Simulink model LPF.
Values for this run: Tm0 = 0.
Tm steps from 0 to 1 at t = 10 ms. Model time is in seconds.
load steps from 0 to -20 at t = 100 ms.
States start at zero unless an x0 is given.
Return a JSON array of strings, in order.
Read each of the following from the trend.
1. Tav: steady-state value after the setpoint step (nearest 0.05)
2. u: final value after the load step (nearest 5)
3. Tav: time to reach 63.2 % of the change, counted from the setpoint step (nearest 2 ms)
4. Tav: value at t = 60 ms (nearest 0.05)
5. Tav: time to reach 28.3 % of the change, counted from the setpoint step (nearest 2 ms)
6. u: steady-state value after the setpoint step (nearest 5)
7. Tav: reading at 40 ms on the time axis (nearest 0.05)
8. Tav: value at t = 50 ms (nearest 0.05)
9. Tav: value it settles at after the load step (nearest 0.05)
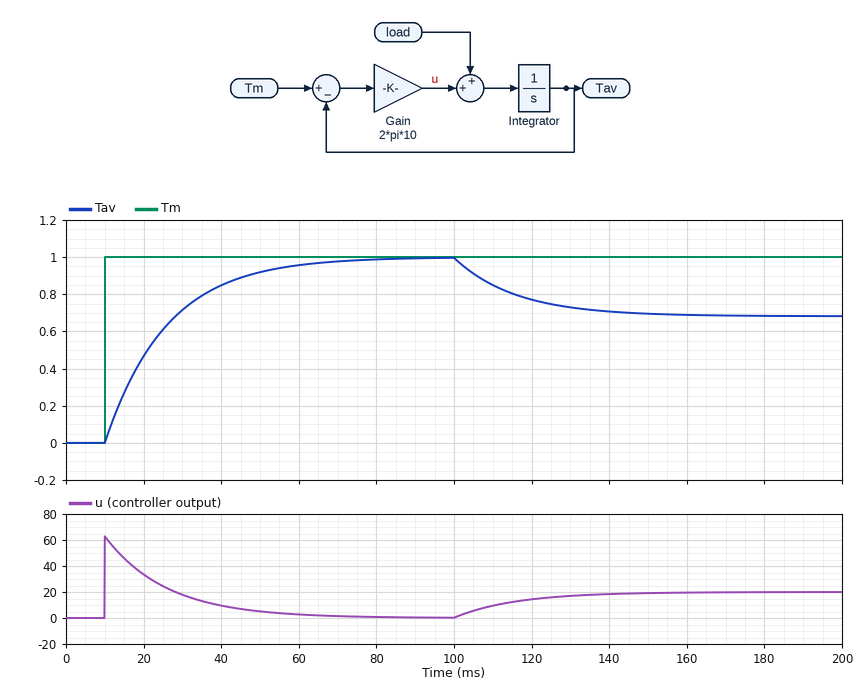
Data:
["1.00", "20", "16 ms", "0.95", "6 ms", "0", "0.85", "0.90", "0.70"]
